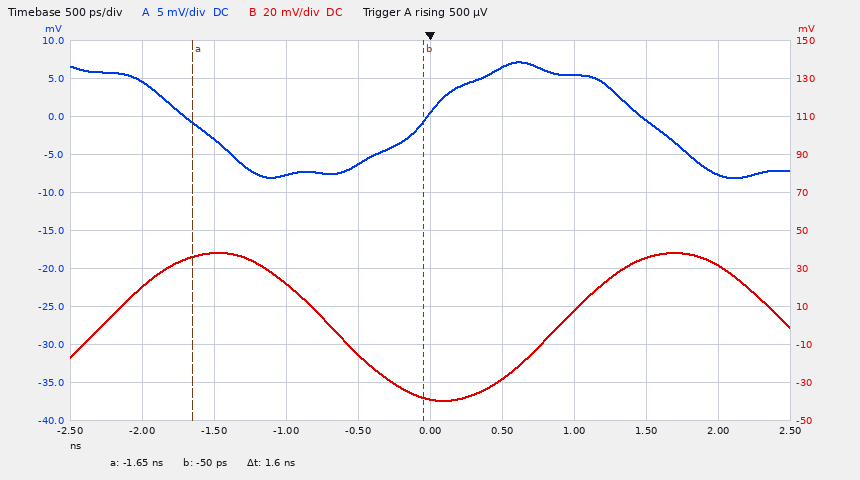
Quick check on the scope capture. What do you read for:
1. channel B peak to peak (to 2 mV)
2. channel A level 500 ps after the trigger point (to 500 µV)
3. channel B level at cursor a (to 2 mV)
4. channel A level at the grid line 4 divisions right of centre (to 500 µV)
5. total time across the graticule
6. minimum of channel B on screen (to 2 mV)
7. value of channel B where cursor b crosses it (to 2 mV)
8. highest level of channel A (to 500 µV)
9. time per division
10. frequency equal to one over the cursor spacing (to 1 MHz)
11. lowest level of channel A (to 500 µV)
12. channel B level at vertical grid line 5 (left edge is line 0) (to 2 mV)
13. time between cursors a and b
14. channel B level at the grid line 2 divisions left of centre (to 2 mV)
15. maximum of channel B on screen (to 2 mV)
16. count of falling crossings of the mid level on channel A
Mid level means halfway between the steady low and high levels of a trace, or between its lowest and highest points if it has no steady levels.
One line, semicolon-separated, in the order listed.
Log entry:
78 mV; 6.5 mV; 36 mV; -7.5 mV; 5 ns; -40 mV; -38 mV; 7.0 mV; 500 ps; 625 MHz; -8.0 mV; -38 mV; 1.6 ns; 22 mV; 38 mV; 2
